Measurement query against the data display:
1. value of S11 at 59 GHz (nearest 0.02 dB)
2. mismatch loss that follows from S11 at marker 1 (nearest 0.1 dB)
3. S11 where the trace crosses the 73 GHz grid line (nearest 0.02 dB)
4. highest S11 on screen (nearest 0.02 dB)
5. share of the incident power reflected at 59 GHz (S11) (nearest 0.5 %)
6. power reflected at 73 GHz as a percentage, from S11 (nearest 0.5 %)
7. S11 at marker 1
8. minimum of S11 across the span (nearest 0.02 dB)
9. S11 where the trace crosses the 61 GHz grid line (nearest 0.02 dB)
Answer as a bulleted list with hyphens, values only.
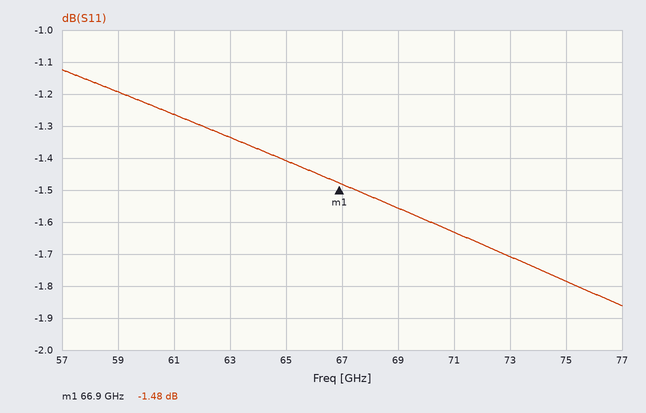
- -1.20 dB
- 5.4 dB
- -1.70 dB
- -1.12 dB
- 76.0 %
- 67.5 %
- -1.48 dB
- -1.86 dB
- -1.26 dB
